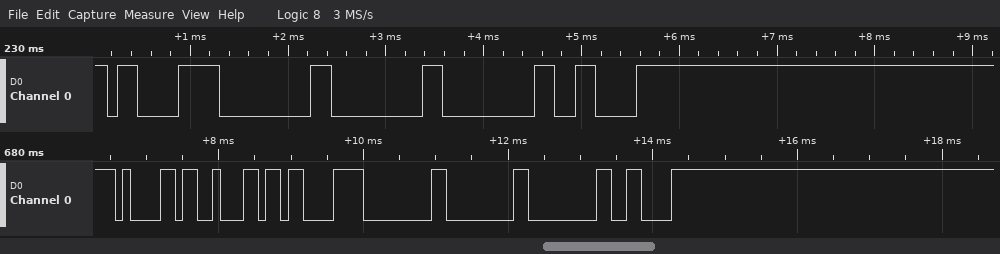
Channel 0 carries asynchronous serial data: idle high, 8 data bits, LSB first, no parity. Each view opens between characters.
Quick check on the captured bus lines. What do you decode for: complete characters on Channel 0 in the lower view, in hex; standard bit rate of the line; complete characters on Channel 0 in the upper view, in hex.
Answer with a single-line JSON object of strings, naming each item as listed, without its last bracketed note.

{"complete characters on Channel 0 in the lower view, in hex": "61, 62, C3, 00, 00, 00, 86", "standard bit rate of the line": "9600 baud", "complete characters on Channel 0 in the upper view, in hex": "C3, 00, 00, 00, 86"}
